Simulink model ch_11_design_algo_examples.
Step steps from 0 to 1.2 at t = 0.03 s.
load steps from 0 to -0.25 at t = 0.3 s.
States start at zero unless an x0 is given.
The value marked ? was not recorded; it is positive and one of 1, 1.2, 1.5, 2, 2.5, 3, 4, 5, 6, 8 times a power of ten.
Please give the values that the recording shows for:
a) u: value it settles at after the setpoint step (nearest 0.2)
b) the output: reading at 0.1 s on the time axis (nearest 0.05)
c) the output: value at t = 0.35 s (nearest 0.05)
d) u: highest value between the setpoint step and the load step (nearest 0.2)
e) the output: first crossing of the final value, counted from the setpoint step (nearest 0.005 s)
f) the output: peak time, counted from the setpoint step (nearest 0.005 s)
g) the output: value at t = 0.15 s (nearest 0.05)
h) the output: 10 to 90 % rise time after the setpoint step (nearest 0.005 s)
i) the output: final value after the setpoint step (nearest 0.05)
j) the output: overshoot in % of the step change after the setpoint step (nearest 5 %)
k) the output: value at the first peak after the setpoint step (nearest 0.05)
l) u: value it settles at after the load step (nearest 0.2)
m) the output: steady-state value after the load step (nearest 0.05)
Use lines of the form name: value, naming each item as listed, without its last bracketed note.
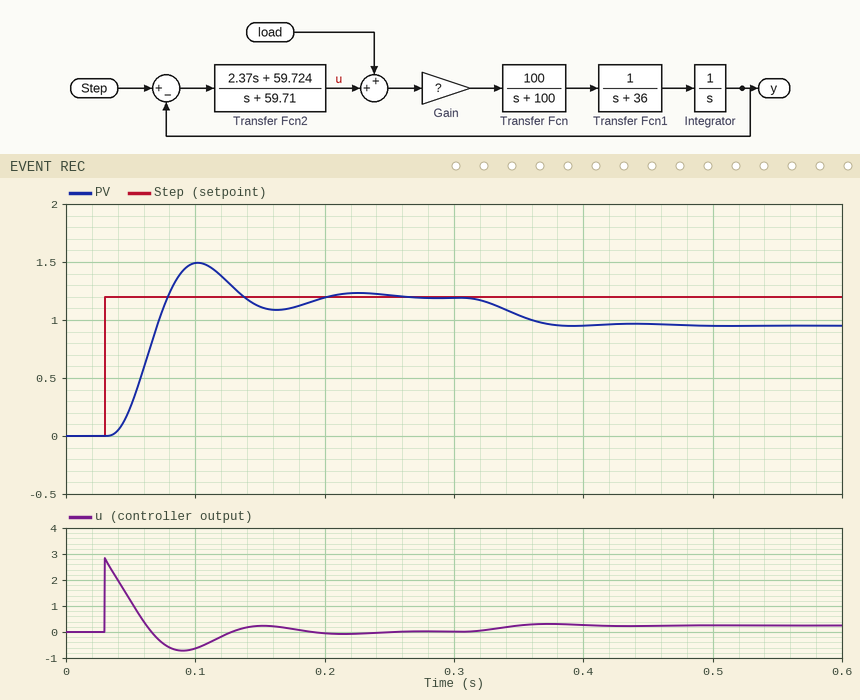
u: value it settles at after the setpoint step: 0.0
the output: reading at 0.1 s on the time axis: 1.50
the output: value at t = 0.35 s: 1.05
u: highest value between the setpoint step and the load step: 2.8
the output: first crossing of the final value, counted from the setpoint step: 0.050 s
the output: peak time, counted from the setpoint step: 0.070 s
the output: value at t = 0.15 s: 1.10
the output: 10 to 90 % rise time after the setpoint step: 0.030 s
the output: final value after the setpoint step: 1.20
the output: overshoot in % of the step change after the setpoint step: 25 %
the output: value at the first peak after the setpoint step: 1.50
u: value it settles at after the load step: 0.2
the output: steady-state value after the load step: 0.95
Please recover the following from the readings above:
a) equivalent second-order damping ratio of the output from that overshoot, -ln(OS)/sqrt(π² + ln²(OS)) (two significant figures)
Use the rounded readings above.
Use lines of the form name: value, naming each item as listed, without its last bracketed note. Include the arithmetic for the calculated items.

equivalent second-order damping ratio of the output from that overshoot, -ln(OS)/sqrt(π² + ln²(OS)): ln(0.25) = -1.386; 1.386 / sqrt(9.870 + 1.922) = 0.40
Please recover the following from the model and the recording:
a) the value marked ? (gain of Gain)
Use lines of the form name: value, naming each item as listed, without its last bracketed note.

the value marked ?: 1500
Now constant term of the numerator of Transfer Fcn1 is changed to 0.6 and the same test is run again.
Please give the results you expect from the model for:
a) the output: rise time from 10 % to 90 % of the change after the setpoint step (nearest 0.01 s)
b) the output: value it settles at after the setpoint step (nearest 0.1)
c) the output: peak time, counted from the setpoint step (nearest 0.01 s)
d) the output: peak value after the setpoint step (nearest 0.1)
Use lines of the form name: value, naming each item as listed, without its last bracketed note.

the output: rise time from 10 % to 90 % of the change after the setpoint step: 0.05 s
the output: value it settles at after the setpoint step: 1.2
the output: peak time, counted from the setpoint step: 0.10 s
the output: peak value after the setpoint step: 1.3
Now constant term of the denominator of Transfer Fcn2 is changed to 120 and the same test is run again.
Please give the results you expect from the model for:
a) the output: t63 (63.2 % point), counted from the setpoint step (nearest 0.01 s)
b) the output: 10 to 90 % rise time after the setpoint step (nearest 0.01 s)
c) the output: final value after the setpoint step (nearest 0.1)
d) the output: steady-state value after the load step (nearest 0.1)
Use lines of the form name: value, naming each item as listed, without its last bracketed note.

the output: t63 (63.2 % point), counted from the setpoint step: 0.05 s
the output: 10 to 90 % rise time after the setpoint step: 0.07 s
the output: final value after the setpoint step: 1.2
the output: steady-state value after the load step: 0.7
